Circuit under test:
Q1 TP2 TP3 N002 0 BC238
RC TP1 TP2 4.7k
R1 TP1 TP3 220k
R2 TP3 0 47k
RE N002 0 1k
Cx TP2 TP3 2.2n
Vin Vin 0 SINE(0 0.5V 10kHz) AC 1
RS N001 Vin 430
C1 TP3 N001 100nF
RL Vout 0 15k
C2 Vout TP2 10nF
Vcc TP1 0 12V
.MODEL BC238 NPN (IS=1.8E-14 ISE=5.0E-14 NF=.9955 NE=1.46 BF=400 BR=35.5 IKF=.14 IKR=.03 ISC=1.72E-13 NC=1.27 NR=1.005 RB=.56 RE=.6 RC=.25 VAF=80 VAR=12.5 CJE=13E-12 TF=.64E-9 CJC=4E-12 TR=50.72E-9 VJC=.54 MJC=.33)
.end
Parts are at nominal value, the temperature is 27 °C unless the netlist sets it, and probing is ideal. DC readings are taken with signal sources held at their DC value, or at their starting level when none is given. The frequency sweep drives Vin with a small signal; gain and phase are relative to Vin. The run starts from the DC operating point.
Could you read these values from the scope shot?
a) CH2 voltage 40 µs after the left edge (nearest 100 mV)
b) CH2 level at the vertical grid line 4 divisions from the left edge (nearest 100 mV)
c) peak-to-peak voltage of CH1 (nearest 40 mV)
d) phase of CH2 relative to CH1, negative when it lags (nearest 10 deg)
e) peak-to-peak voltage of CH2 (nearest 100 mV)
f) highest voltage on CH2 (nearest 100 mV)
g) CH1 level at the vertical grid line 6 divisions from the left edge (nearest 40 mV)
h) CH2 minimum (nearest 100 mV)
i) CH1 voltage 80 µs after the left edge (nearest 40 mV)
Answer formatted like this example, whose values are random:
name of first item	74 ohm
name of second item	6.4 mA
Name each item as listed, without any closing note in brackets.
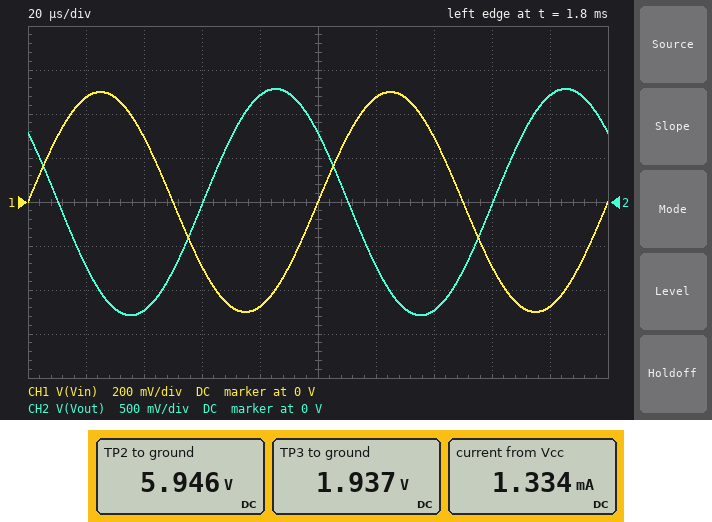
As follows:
CH2 voltage 40 µs after the left edge	-1.2 V
CH2 level at the vertical grid line 4 divisions from the left edge	1.2 V
peak-to-peak voltage of CH1	1.00 V
phase of CH2 relative to CH1, negative when it lags	140 deg
peak-to-peak voltage of CH2	2.6 V
highest voltage on CH2	1.3 V
CH1 level at the vertical grid line 6 divisions from the left edge	480 mV
CH2 minimum	-1.3 V
CH1 voltage 80 µs after the left edge	-480 mV
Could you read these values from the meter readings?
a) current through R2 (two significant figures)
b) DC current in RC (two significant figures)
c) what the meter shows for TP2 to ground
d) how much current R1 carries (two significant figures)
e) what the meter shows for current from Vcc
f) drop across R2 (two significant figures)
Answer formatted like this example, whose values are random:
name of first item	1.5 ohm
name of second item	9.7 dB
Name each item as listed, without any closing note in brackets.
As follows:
current through R2	41 µA
DC current in RC	1.3 mA
what the meter shows for TP2 to ground	5.946 V
how much current R1 carries	46 µA
what the meter shows for current from Vcc	1.334 mA
drop across R2	1.9 V
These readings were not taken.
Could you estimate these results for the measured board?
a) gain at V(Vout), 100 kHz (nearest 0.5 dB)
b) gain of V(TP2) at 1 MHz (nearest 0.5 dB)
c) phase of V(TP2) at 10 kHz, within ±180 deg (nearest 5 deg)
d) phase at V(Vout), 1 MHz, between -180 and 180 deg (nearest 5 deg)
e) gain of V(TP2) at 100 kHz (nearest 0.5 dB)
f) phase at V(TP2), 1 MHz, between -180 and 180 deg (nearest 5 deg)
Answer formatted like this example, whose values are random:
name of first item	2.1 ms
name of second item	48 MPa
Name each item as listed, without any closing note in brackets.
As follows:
gain at V(Vout), 100 kHz	-2.0 dB
gain of V(TP2) at 1 MHz	-4.0 dB
phase of V(TP2) at 10 kHz, within ±180 deg	135 deg
phase at V(Vout), 1 MHz, between -180 and 180 deg	5 deg
gain of V(TP2) at 100 kHz	-2.0 dB
phase at V(TP2), 1 MHz, between -180 and 180 deg	5 deg
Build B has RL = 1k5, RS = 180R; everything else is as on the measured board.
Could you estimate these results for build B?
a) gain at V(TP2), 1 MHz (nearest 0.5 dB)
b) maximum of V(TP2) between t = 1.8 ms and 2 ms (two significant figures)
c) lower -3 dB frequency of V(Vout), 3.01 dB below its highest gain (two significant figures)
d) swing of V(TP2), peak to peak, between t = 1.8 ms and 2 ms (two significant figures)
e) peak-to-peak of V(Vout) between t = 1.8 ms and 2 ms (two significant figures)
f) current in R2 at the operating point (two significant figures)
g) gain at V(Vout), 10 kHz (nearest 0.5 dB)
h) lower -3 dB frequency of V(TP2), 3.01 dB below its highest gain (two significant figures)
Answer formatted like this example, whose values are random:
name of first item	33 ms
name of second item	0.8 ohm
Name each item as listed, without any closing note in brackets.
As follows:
gain at V(TP2), 1 MHz	-2.5 dB
maximum of V(TP2) between t = 1.8 ms and 2 ms	6.6 V
lower -3 dB frequency of V(Vout), 3.01 dB below its highest gain	2.3 kHz
swing of V(TP2), peak to peak, between t = 1.8 ms and 2 ms	1.3 V
peak-to-peak of V(Vout) between t = 1.8 ms and 2 ms	890 mV
current in R2 at the operating point	41 µA
gain at V(Vout), 10 kHz	-1.0 dB
lower -3 dB frequency of V(TP2), 3.01 dB below its highest gain	40 Hz
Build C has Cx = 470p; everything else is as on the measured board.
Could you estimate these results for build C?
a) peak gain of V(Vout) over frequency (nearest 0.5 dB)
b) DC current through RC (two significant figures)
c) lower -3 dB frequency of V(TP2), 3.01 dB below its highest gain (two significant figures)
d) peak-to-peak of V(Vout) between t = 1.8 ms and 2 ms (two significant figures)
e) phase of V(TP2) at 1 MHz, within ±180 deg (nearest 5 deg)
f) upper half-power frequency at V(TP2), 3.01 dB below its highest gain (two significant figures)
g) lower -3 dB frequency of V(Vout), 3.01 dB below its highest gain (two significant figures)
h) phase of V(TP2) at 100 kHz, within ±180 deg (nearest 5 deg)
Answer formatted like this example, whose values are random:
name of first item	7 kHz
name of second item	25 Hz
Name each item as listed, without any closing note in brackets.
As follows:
peak gain of V(Vout) over frequency	10.5 dB
DC current through RC	1.3 mA
lower -3 dB frequency of V(TP2), 3.01 dB below its highest gain	42 Hz
peak-to-peak of V(Vout) between t = 1.8 ms and 2 ms	3.3 V
phase of V(TP2) at 1 MHz, within ±180 deg	20 deg
upper half-power frequency at V(TP2), 3.01 dB below its highest gain	32 kHz
lower -3 dB frequency of V(Vout), 3.01 dB below its highest gain	790 Hz
phase of V(TP2) at 100 kHz, within ±180 deg	105 deg
